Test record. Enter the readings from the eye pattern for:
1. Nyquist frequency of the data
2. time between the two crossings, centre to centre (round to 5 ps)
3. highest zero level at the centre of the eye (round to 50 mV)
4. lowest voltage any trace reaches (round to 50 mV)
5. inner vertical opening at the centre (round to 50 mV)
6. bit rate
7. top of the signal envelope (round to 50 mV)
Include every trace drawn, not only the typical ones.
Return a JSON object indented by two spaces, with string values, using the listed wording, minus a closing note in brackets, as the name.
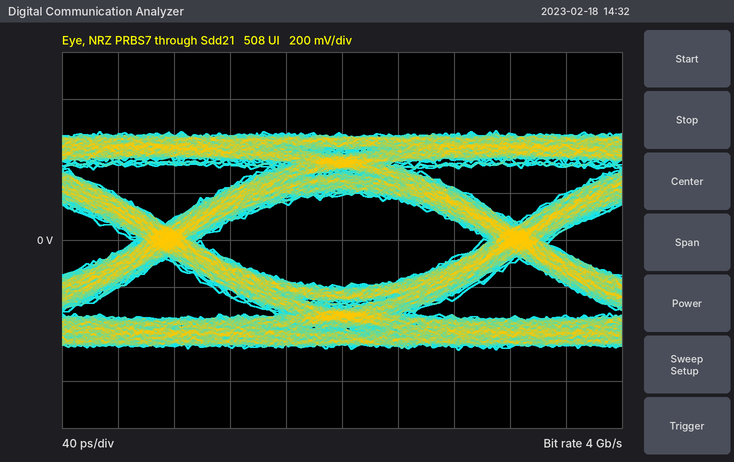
{
  "Nyquist frequency of the data": "2 GHz",
  "time between the two crossings, centre to centre": "250 ps",
  "highest zero level at the centre of the eye": "-200 mV",
  "lowest voltage any trace reaches": "-450 mV",
  "inner vertical opening at the centre": "400 mV",
  "bit rate": "4 Gb/s",
  "top of the signal envelope": "450 mV"
}
